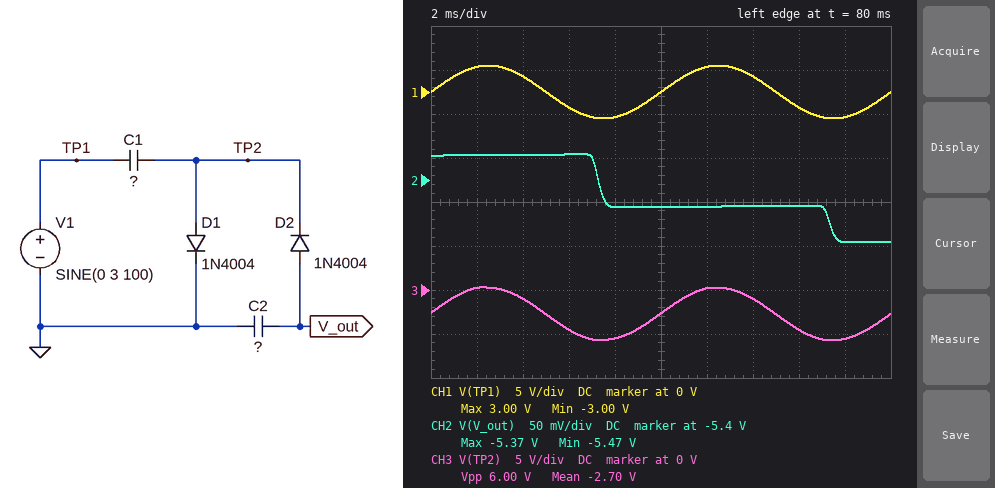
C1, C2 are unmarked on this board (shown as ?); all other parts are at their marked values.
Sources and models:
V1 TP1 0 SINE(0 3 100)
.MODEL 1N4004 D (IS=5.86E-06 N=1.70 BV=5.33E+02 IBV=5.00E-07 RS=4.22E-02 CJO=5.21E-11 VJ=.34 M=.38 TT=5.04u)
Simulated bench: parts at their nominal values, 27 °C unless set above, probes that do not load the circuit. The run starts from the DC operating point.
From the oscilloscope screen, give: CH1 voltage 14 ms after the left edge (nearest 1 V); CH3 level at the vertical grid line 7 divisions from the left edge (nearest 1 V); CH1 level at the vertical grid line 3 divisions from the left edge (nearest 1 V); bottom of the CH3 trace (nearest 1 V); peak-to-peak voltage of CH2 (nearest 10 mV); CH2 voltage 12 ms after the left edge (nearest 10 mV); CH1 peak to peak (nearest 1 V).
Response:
2 V
-1 V
-2 V
-6 V
100 mV
-5.43 V
6 V
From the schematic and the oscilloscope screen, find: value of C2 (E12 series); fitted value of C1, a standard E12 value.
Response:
27 µF
15 µF
